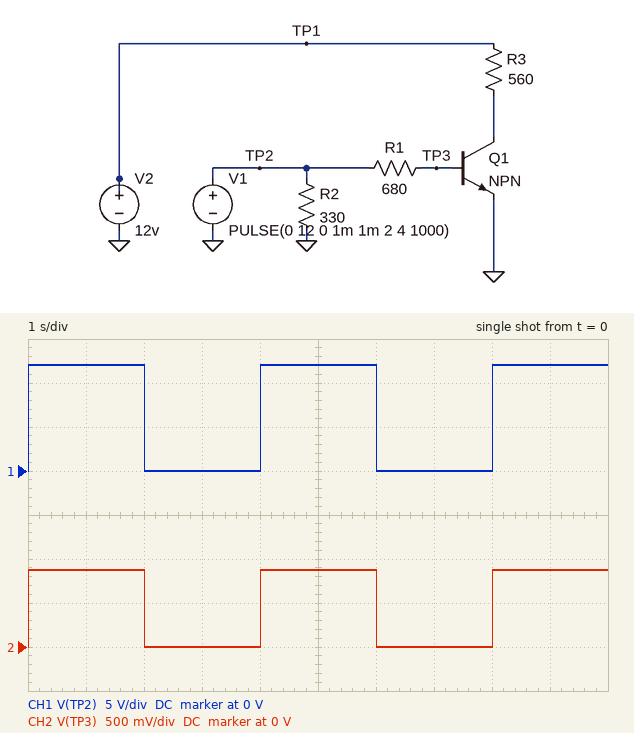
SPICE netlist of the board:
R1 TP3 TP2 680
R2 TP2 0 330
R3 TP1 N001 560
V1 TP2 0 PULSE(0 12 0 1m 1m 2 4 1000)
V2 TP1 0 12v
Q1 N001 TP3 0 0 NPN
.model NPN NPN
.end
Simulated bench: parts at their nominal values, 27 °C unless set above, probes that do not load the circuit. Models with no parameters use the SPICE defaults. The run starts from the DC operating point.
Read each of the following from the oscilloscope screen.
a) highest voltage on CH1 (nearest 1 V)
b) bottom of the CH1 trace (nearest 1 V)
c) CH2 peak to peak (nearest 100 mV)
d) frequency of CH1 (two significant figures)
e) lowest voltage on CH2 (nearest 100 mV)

12 V
0 V
900 mV
250 mHz
0 V
